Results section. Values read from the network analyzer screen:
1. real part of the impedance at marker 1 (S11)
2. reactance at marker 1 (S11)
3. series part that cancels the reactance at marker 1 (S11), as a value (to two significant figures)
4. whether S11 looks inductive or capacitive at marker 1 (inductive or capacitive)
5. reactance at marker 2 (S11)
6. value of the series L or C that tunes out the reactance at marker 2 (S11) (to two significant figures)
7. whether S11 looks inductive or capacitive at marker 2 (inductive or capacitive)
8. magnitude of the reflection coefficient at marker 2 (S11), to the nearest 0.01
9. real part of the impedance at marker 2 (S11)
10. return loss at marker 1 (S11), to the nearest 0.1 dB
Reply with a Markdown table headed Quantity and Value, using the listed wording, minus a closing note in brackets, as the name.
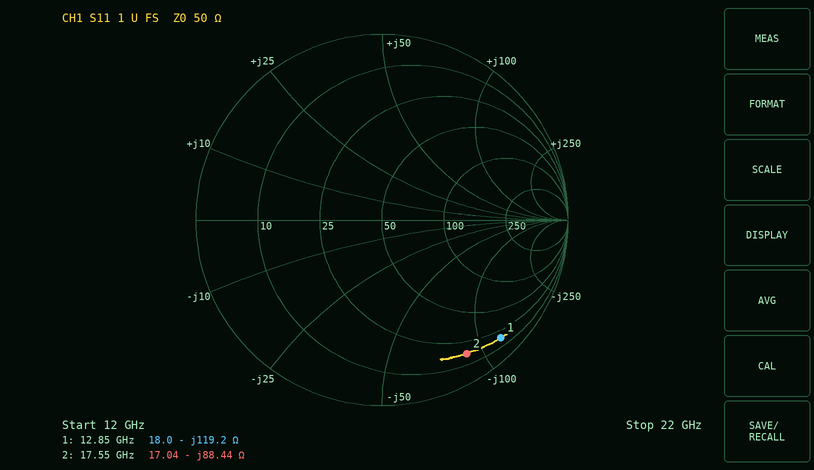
| Quantity | Value |
|---|---|
| real part of the impedance at marker 1 | 18.0 Ω |
| reactance at marker 1 | -119.2 Ω |
| series part that cancels the reactance at marker 1 (S11), as a value | 1.5 nH |
| whether S11 looks inductive or capacitive at marker 1 | capacitive |
| reactance at marker 2 | -88.44 Ω |
| value of the series L or C that tunes out the reactance at marker 2 (S11) | 800 pH |
| whether S11 looks inductive or capacitive at marker 2 | capacitive |
| magnitude of the reflection coefficient at marker 2 (S11), to the nearest 0.01 | 0.85 |
| real part of the impedance at marker 2 | 17.04 Ω |
| return loss at marker 1 (S11), to the nearest 0.1 dB | 0.9 dB |
